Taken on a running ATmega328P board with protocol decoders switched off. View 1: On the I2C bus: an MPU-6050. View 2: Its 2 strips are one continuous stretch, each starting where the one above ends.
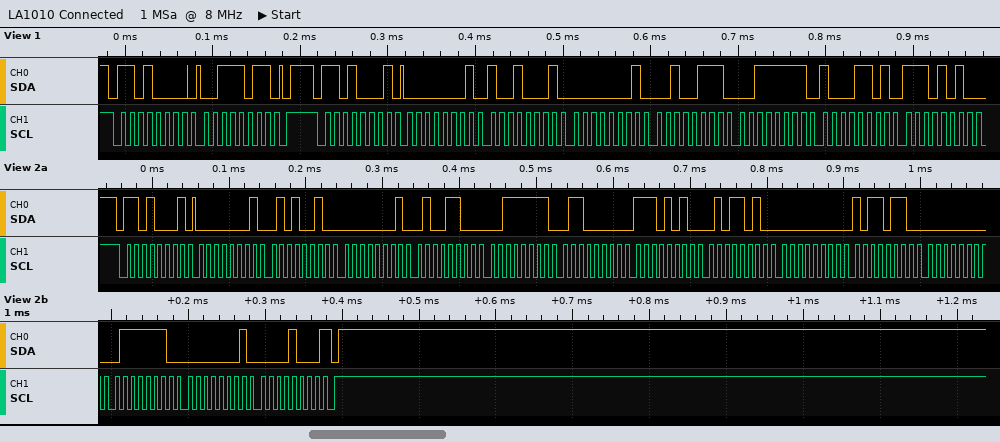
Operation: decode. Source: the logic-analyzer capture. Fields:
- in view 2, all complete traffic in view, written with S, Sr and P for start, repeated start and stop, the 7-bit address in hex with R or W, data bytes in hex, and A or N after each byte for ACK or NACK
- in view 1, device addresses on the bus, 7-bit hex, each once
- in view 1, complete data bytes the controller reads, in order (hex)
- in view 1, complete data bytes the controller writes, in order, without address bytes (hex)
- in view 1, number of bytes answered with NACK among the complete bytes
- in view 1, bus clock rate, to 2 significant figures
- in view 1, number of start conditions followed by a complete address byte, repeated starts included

S 68R A 01 A 52 A 01 A 4C A 3F A 60 A EA A 5A A 00 A B6 A 00 A 7E A 01 A 08 N P
0x68
01 91 01 27 3F 8D EA
3B
0
100 kHz
2
